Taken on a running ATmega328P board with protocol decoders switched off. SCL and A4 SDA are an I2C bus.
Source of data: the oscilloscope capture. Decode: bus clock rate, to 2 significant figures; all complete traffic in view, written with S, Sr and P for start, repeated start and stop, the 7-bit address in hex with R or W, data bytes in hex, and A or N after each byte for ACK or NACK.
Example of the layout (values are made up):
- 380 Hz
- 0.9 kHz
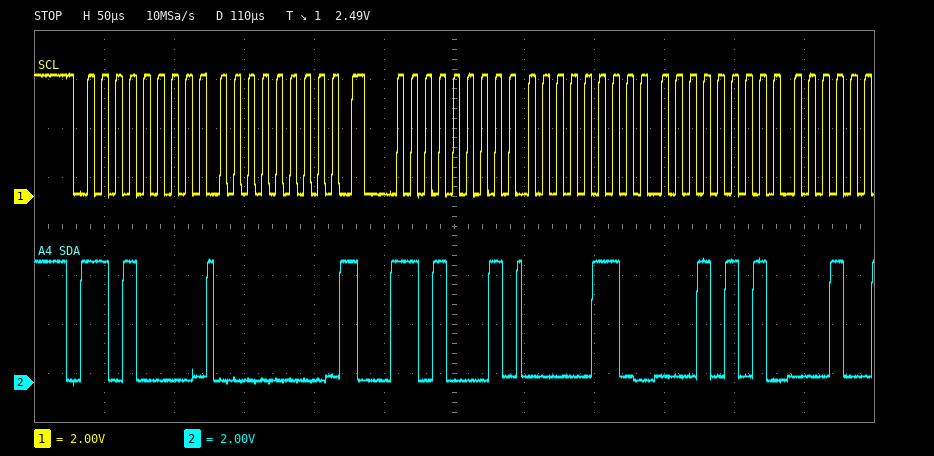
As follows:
- 100 kHz
- S 68W A 00 A Sr 68R A 06 A 15 A
